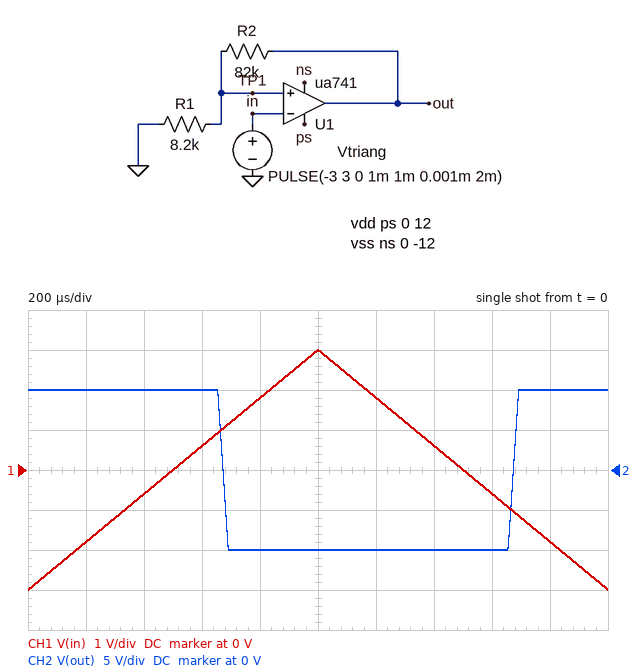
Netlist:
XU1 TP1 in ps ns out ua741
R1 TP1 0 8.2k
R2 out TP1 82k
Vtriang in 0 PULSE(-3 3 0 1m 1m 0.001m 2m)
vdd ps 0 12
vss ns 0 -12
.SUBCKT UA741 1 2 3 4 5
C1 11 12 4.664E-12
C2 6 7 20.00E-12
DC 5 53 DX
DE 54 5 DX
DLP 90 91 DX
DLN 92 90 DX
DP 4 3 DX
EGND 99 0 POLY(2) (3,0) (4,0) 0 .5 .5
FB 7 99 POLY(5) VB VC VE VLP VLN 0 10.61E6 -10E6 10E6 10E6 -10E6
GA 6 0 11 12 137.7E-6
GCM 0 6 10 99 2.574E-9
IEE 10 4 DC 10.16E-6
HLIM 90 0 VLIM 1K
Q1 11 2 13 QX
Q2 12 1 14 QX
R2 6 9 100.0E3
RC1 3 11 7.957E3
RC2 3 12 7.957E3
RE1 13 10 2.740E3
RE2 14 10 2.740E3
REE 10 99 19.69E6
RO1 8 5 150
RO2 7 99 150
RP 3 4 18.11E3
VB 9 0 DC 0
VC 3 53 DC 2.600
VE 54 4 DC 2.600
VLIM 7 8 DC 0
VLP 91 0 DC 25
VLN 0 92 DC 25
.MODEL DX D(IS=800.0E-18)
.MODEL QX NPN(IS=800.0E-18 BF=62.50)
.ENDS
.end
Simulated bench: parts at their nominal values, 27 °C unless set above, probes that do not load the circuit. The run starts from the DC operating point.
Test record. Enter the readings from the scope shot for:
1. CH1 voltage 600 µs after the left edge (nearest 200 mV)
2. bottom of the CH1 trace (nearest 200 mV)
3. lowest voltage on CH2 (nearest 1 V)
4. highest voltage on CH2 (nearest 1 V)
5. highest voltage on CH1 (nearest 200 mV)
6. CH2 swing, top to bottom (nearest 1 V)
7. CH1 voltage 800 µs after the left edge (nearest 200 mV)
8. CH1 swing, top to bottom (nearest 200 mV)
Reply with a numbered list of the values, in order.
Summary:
1. 600 mV
2. -3.0 V
3. -10 V
4. 10 V
5. 3.0 V
6. 20 V
7. 1.8 V
8. 6.0 V
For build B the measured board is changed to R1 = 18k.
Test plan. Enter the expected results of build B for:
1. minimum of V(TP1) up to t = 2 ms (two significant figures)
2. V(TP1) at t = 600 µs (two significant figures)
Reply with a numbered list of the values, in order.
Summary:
1. -1.8 V
2. 1.8 V
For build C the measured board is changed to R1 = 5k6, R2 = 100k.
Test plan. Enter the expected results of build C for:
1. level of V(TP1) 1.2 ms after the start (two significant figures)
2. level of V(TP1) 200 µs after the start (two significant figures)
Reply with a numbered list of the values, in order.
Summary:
1. -530 mV
2. 530 mV
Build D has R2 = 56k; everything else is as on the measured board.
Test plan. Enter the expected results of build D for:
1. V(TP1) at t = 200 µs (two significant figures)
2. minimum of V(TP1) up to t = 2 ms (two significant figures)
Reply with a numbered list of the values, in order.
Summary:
1. 1.3 V
2. -1.3 V
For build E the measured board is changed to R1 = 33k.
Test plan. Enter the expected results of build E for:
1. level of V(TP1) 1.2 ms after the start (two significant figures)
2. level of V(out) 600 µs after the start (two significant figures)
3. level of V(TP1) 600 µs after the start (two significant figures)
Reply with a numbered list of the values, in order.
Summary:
1. -2.9 V
2. 10 V
3. 2.9 V
